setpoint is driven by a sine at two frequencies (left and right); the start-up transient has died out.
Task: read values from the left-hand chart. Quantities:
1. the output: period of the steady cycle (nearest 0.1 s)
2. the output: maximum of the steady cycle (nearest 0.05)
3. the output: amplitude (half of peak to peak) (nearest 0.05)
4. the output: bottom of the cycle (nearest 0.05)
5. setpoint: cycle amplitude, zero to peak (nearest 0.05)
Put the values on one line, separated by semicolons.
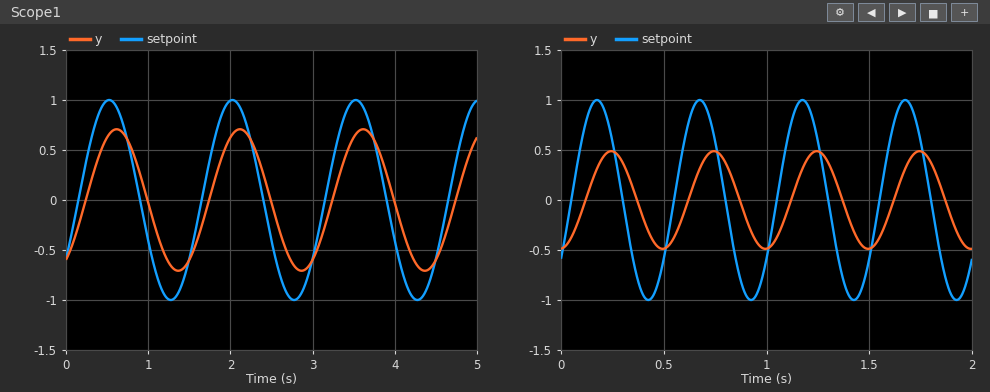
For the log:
1.5 s; 0.70; 0.70; -0.70; 1.00
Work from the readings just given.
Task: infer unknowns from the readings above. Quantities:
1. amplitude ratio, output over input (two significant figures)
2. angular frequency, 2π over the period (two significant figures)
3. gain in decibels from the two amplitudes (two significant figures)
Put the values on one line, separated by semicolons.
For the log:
0.70; 4.2 rad/s; -3.1 dB
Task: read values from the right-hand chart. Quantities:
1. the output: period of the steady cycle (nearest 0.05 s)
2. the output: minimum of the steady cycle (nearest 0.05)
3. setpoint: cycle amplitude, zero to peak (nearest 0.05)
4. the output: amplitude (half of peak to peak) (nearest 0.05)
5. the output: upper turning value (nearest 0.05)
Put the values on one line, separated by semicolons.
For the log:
0.50 s; -0.50; 1.00; 0.50; 0.50
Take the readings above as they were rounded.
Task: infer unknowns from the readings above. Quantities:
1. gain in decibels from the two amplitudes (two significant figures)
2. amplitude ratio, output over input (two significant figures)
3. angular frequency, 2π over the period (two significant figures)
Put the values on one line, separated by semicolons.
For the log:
-6.0 dB; 0.50; 13 rad/s
